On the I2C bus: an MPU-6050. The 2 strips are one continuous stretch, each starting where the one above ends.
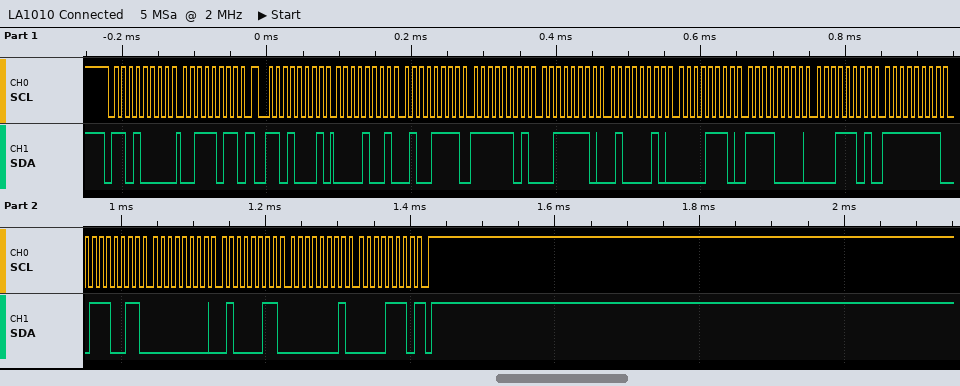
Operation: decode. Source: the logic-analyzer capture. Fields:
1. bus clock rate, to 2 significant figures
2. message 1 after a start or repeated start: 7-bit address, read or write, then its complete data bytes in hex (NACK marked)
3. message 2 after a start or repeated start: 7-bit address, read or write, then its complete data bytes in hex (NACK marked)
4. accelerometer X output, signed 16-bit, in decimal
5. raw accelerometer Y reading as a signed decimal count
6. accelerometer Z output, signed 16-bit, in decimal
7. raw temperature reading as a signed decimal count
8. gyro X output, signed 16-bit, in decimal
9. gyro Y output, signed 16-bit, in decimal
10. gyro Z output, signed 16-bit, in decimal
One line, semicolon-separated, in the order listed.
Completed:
100 kHz; 0x68 write: 3B; 0x68 read: 09 4F FD 3E 42 0E F0 1D FF 73 00 43 01 0E NACK; 2383; -706; 16910; -4067; -141; 67; 270
